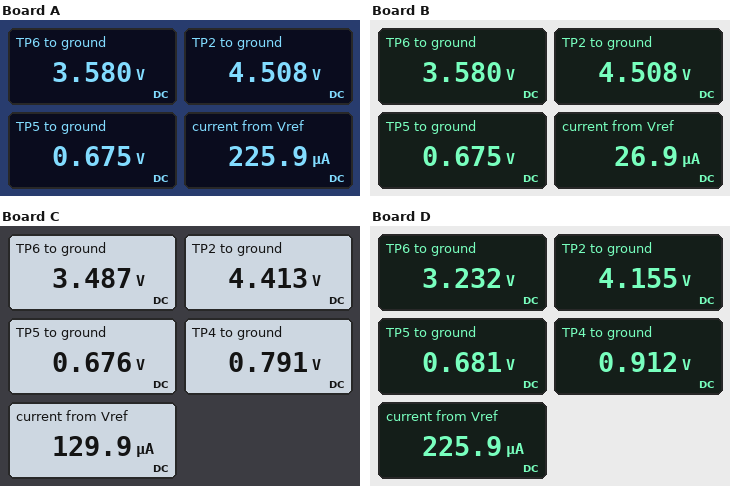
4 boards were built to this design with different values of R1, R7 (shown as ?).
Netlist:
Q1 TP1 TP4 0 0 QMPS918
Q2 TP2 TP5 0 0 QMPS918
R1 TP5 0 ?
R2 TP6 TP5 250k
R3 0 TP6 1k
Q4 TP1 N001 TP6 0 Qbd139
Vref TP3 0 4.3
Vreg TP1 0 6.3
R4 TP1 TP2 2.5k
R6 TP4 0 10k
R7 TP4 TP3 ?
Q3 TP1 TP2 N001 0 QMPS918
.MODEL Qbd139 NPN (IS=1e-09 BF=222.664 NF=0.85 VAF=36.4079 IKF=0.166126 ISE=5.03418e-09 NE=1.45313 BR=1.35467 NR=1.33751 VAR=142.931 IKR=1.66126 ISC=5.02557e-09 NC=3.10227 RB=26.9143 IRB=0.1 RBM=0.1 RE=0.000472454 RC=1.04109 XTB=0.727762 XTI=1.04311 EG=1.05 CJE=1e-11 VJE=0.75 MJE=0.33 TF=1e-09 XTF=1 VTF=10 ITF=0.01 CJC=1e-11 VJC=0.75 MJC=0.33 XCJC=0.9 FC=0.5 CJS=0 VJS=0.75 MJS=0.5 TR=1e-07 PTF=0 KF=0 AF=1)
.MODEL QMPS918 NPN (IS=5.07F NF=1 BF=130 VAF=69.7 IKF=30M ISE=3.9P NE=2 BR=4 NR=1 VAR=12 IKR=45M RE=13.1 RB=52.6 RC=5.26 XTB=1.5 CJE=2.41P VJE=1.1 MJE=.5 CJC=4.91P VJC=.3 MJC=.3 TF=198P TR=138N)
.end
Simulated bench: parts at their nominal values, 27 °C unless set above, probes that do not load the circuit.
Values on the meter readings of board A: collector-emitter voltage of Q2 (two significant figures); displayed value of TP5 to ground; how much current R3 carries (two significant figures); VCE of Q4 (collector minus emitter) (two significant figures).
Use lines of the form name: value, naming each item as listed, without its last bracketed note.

collector-emitter voltage of Q2: 4.5 V
displayed value of TP5 to ground: 0.675 V
how much current R3 carries: 3.6 mA
VCE of Q4 (collector minus emitter): 2.7 V
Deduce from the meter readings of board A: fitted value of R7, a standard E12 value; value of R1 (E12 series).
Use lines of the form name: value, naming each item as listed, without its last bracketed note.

fitted value of R7, a standard E12 value: 15 kΩ
value of R1: 150 kΩ
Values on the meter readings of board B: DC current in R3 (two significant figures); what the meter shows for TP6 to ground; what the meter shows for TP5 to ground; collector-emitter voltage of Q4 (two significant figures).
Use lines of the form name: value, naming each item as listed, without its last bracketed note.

DC current in R3: 3.6 mA
what the meter shows for TP6 to ground: 3.580 V
what the meter shows for TP5 to ground: 0.675 V
collector-emitter voltage of Q4: 2.7 V
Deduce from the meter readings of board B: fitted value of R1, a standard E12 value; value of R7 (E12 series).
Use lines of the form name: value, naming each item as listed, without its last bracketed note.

fitted value of R1, a standard E12 value: 150 kΩ
value of R7: 150 kΩ
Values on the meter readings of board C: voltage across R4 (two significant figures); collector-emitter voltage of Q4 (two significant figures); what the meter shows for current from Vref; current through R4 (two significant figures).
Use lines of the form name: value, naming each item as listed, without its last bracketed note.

voltage across R4: 1.9 V
collector-emitter voltage of Q4: 2.8 V
what the meter shows for current from Vref: 129.9 µA
current through R4: 750 µA
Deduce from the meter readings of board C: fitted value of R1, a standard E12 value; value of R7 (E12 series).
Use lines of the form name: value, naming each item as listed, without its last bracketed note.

fitted value of R1, a standard E12 value: 180 kΩ
value of R7: 27 kΩ
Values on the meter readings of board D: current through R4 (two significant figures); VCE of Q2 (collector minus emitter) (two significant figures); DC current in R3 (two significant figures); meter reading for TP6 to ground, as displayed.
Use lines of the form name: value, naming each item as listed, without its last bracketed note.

current through R4: 860 µA
VCE of Q2 (collector minus emitter): 4.2 V
DC current in R3: 3.2 mA
meter reading for TP6 to ground, as displayed: 3.232 V
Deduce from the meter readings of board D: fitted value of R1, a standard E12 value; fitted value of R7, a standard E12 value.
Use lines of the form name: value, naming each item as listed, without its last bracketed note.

fitted value of R1, a standard E12 value: 390 kΩ
fitted value of R7, a standard E12 value: 15 kΩ
